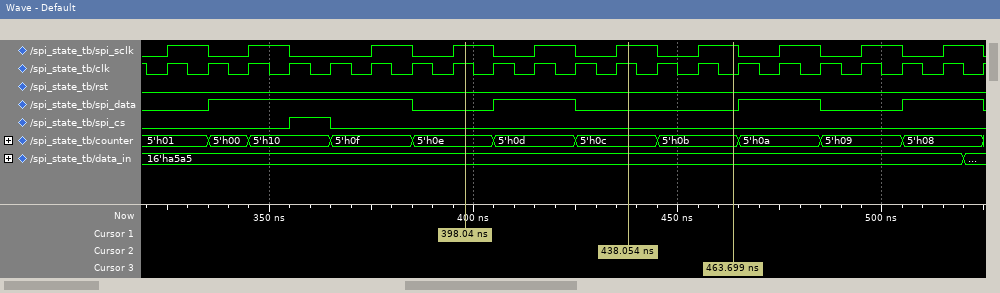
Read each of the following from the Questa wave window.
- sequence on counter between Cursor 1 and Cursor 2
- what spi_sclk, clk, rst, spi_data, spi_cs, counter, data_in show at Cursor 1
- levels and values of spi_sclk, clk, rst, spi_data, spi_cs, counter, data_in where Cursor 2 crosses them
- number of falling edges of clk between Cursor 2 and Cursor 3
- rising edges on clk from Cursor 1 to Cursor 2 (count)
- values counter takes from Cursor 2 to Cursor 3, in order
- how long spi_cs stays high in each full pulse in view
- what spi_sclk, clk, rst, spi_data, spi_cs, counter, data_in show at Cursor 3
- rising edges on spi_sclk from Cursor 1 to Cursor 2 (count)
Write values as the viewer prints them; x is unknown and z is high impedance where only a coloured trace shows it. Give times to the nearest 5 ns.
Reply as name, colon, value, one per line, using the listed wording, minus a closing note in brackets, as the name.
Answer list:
sequence on counter between Cursor 1 and Cursor 2: 5'h0e, 5'h0d, 5'h0c
what spi_sclk, clk, rst, spi_data, spi_cs, counter, data_in show at Cursor 1: spi_sclk=1, clk=1, rst=0, spi_data=0, spi_cs=0, counter=5'h0e, data_in=16'ha5a5
levels and values of spi_sclk, clk, rst, spi_data, spi_cs, counter, data_in where Cursor 2 crosses them: spi_sclk=1, clk=1, rst=0, spi_data=0, spi_cs=0, counter=5'h0c, data_in=16'ha5a5
number of falling edges of clk between Cursor 2 and Cursor 3: 3
rising edges on clk from Cursor 1 to Cursor 2: 4
values counter takes from Cursor 2 to Cursor 3, in order: 5'h0c, 5'h0b
how long spi_cs stays high in each full pulse in view: 10 ns
what spi_sclk, clk, rst, spi_data, spi_cs, counter, data_in show at Cursor 3: spi_sclk=1, clk=0, rst=0, spi_data=0, spi_cs=0, counter=5'h0b, data_in=16'ha5a5
rising edges on spi_sclk from Cursor 1 to Cursor 2: 2
